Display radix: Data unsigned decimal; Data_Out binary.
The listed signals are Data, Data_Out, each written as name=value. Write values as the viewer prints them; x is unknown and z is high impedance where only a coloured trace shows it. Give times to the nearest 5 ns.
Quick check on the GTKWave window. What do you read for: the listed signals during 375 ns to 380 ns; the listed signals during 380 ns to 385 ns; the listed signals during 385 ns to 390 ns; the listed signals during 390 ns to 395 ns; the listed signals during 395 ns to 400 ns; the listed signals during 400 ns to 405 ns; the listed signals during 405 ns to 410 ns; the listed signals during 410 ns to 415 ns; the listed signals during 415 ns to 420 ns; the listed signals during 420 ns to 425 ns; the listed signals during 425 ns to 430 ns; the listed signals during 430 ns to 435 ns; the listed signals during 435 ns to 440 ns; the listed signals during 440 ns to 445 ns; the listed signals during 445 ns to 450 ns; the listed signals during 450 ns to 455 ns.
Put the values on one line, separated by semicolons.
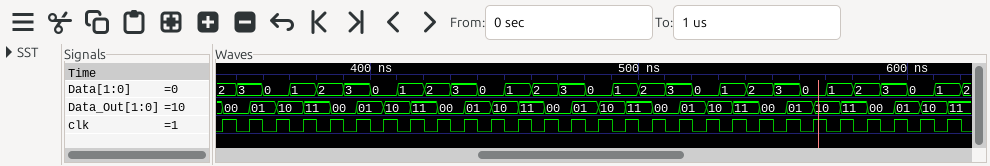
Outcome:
Data=1, Data_Out=11; Data=2, Data_Out=11; Data=2, Data_Out=00; Data=3, Data_Out=00; Data=3, Data_Out=01; Data=0, Data_Out=01; Data=0, Data_Out=10; Data=1, Data_Out=10; Data=1, Data_Out=11; Data=2, Data_Out=11; Data=2, Data_Out=00; Data=3, Data_Out=00; Data=3, Data_Out=01; Data=0, Data_Out=01; Data=0, Data_Out=10; Data=1, Data_Out=10
